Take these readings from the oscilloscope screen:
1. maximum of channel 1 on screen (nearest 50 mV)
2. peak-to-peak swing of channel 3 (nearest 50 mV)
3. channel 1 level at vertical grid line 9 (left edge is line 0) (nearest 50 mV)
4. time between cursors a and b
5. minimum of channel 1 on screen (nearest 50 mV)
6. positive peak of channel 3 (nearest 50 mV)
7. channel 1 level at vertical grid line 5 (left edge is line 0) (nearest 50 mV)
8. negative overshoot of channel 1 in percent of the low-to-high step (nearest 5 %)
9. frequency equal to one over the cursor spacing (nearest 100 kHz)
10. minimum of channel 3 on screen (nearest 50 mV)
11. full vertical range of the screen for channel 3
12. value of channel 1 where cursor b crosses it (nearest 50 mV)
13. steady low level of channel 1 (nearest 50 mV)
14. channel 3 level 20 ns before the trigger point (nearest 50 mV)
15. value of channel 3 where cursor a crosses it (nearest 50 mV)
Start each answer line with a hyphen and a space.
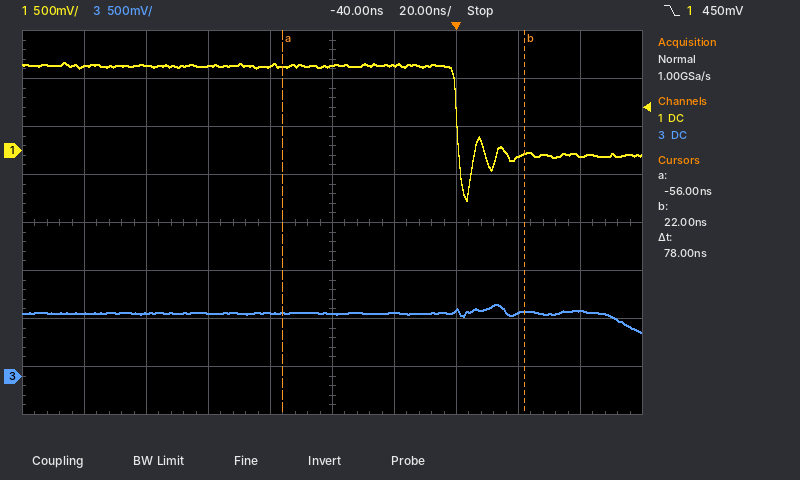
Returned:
- 900 mV
- 300 mV
- -50 mV
- 78 ns
- -500 mV
- 750 mV
- 900 mV
- 50 %
- 12.8 MHz
- 450 mV
- 4 V
- -50 mV
- -50 mV
- 650 mV
- 650 mV
